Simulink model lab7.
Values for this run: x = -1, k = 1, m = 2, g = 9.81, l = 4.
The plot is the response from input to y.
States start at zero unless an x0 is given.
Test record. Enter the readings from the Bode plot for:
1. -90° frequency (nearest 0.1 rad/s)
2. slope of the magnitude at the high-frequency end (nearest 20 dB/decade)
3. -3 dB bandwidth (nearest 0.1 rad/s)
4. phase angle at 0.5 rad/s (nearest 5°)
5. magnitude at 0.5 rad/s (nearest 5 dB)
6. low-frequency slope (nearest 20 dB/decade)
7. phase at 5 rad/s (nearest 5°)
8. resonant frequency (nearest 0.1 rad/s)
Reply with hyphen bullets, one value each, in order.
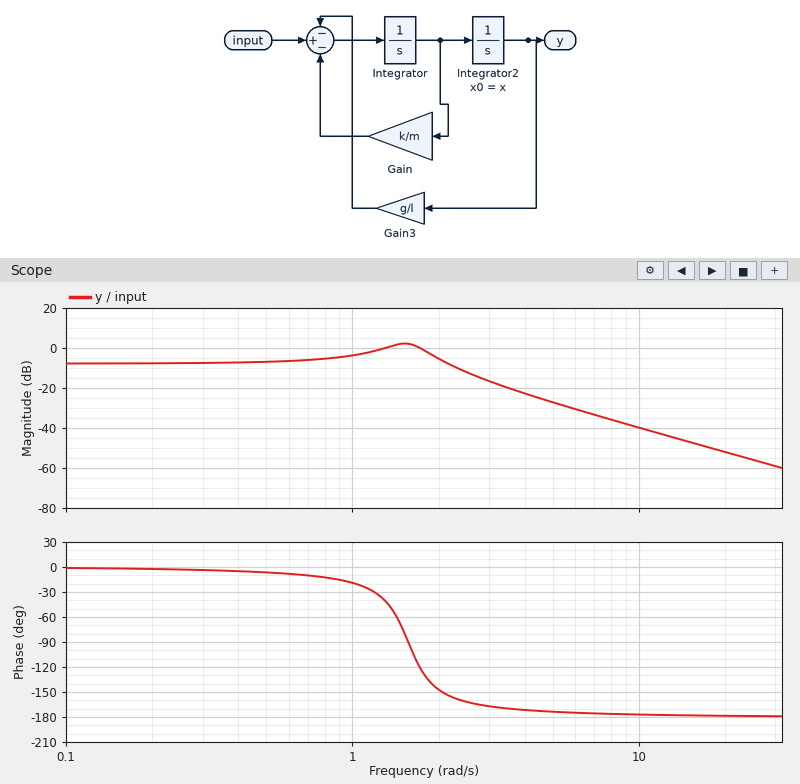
- 1.6 rad/s
- -40 dB/decade
- 2.4 rad/s
- -5°
- -5 dB
- 0 dB/decade
- -175°
- 1.5 rad/s
